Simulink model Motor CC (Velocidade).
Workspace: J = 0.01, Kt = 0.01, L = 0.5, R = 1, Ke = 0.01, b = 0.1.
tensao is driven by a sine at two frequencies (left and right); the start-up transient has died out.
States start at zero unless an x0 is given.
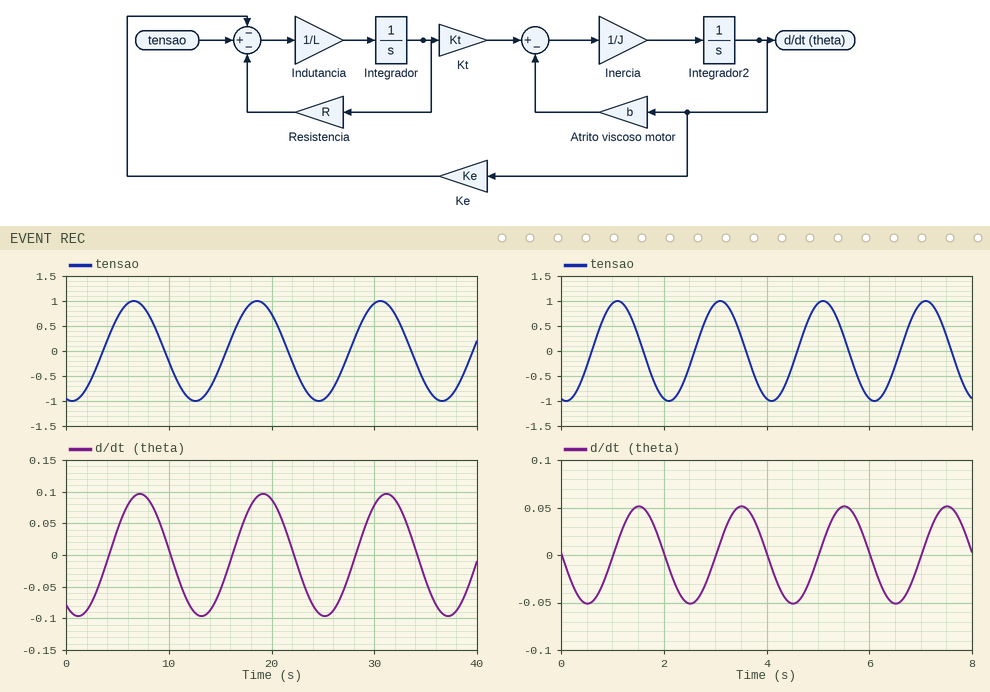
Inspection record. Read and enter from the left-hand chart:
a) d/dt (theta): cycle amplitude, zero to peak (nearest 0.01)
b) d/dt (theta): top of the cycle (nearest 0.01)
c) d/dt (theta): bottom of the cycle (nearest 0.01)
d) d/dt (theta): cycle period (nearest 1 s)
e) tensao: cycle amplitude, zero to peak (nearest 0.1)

0.10
0.10
-0.10
12 s
1.0
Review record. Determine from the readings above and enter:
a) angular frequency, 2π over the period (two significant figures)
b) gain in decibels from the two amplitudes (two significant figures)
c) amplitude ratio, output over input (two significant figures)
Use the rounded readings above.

0.52 rad/s
-20 dB
0.10
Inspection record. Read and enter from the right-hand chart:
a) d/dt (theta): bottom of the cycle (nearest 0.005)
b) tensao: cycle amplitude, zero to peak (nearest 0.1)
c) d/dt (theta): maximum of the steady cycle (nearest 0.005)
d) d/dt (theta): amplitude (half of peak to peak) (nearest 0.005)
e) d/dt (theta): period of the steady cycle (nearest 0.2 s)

-0.050
1.0
0.050
0.050
2.0 s
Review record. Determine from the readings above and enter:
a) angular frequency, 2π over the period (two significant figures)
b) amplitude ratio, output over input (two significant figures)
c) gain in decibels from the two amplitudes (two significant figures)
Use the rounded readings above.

3.1 rad/s
0.050
-26 dB
